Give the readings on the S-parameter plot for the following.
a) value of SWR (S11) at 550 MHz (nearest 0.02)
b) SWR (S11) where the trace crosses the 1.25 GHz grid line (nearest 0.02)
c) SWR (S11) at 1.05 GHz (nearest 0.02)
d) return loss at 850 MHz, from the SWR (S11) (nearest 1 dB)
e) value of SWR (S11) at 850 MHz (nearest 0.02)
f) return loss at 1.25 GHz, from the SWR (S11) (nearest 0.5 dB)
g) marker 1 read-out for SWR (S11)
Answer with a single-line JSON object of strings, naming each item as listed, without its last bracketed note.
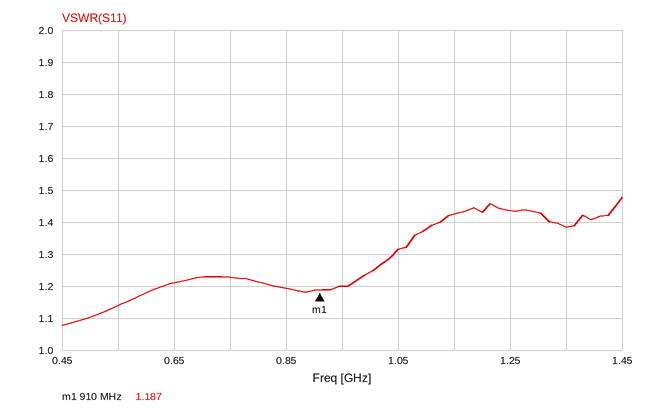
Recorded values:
{"value of SWR (S11) at 550 MHz": "1.14", "SWR (S11) where the trace crosses the 1.25 GHz grid line": "1.44", "SWR (S11) at 1.05 GHz": "1.32", "return loss at 850 MHz, from the SWR (S11)": "21 dB", "value of SWR (S11) at 850 MHz": "1.20", "return loss at 1.25 GHz, from the SWR (S11)": "15.0 dB", "marker 1 read-out for SWR": "1.187"}
